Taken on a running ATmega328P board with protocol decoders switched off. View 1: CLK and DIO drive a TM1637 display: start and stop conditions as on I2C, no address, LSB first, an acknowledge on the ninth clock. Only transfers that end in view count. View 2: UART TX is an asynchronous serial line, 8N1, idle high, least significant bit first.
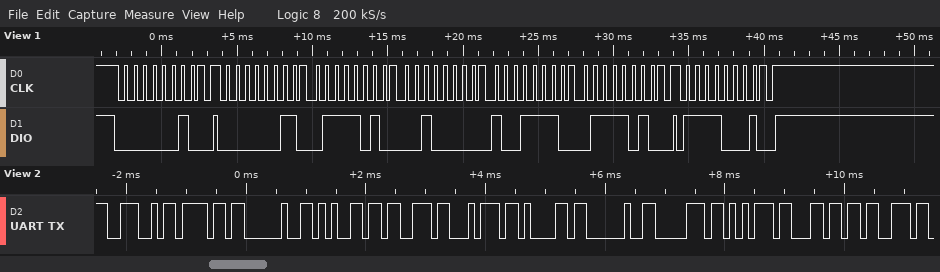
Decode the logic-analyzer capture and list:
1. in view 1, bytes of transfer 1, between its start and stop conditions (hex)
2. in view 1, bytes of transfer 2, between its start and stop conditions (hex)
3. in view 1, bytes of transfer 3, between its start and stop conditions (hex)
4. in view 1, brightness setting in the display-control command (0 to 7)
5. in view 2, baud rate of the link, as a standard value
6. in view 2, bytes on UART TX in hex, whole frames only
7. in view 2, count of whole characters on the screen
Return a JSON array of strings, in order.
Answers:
["40", "C0 5E 04 79 5E", "8F", "7", "9600 baud", "4E 6F 20 65 73 74 61 20 70 75 6C 73", "12"]
